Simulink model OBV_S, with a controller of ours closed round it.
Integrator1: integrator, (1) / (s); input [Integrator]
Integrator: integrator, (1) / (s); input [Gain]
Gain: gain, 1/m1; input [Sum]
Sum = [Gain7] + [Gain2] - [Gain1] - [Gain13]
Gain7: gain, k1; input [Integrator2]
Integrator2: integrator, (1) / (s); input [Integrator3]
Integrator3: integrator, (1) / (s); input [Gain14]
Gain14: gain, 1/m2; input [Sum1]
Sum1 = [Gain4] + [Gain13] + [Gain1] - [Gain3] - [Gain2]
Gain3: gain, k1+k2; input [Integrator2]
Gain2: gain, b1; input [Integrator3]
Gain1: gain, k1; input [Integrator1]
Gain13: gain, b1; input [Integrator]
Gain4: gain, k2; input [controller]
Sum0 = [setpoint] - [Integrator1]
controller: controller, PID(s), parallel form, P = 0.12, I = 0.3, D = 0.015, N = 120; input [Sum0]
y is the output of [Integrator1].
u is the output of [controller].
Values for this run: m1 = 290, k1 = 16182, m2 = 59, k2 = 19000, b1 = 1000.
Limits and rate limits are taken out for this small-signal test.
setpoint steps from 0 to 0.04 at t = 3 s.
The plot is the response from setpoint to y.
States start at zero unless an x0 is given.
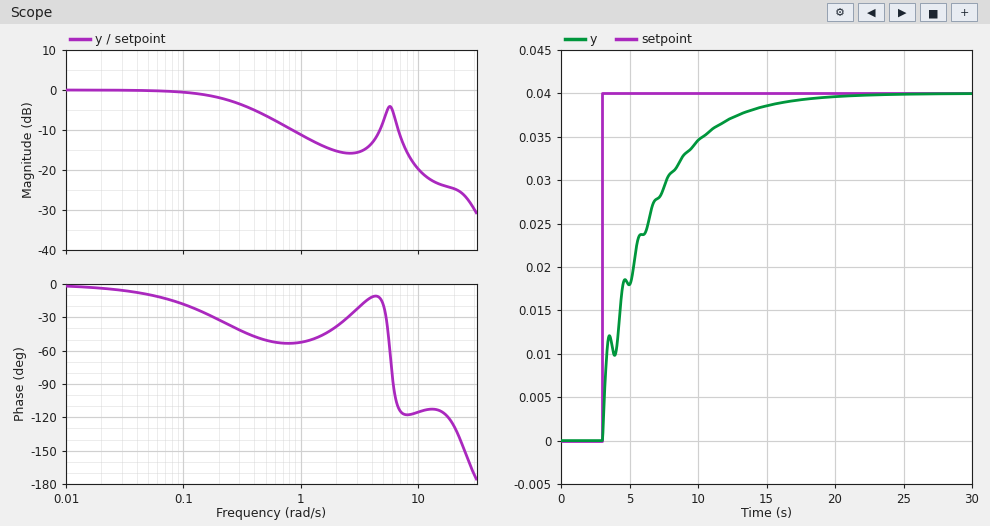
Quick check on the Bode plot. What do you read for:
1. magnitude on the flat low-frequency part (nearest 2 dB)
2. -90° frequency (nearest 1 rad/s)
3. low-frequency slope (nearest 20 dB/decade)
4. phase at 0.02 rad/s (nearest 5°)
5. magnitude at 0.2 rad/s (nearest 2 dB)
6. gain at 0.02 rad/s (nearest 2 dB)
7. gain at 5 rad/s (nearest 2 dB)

0 dB
6 rad/s
0 dB/decade
-5°
-2 dB
0 dB
-8 dB
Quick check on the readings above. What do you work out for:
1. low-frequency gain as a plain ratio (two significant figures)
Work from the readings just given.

1.0
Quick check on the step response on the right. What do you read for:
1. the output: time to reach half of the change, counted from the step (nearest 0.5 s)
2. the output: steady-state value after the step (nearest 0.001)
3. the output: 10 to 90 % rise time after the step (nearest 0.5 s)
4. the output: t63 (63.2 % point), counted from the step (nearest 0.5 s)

2.5 s
0.040
8.0 s
3.5 s
